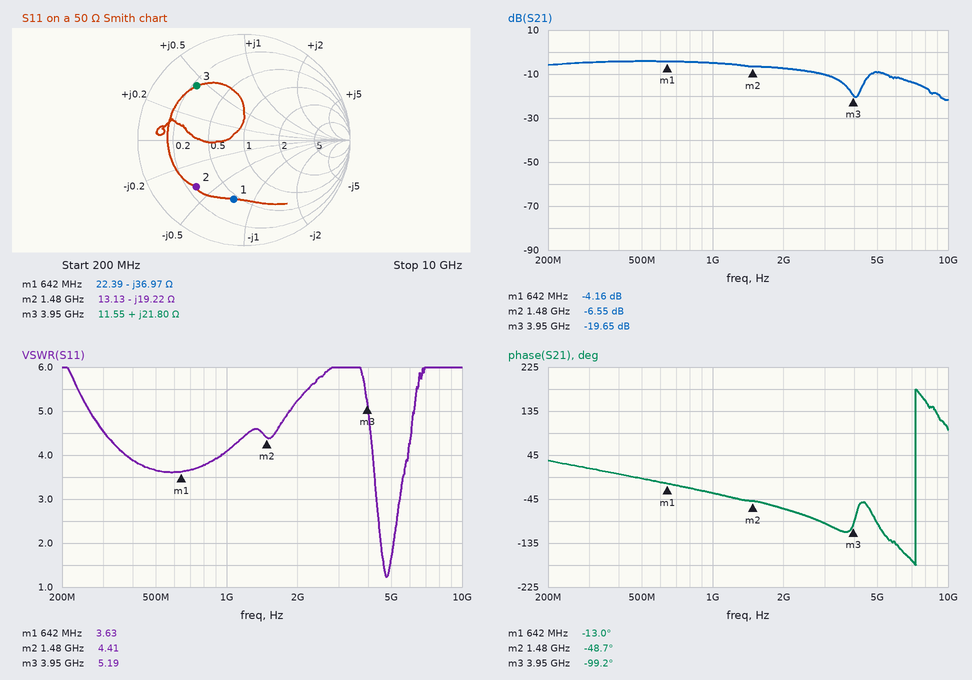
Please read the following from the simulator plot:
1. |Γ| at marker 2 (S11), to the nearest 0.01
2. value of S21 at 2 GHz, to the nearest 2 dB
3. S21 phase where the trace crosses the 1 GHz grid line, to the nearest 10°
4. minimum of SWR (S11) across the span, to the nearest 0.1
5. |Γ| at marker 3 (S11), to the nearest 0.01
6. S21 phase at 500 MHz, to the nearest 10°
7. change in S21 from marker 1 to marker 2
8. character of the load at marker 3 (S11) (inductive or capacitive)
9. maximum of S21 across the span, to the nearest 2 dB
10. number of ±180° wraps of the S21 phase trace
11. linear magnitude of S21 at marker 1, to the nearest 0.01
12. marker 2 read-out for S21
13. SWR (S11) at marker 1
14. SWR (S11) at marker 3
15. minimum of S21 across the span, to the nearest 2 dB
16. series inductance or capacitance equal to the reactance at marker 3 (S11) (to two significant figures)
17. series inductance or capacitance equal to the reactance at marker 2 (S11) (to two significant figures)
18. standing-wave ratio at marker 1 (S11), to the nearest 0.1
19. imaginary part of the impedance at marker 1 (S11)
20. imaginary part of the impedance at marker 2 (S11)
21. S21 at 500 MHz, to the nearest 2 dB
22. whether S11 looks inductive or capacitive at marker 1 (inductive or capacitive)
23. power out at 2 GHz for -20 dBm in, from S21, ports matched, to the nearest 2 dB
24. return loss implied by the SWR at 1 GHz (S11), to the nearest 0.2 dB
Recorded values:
0.63
-8 dB
-30°
1.2
0.68
0°
-2.39 dB
inductive
-4 dB
1
0.62
-6.55 dB
3.63
5.19
-22 dB
880 pH
5.6 pF
3.6
-36.97 Ω
-19.22 Ω
-4 dB
capacitive
-28 dBm
4.4 dB
